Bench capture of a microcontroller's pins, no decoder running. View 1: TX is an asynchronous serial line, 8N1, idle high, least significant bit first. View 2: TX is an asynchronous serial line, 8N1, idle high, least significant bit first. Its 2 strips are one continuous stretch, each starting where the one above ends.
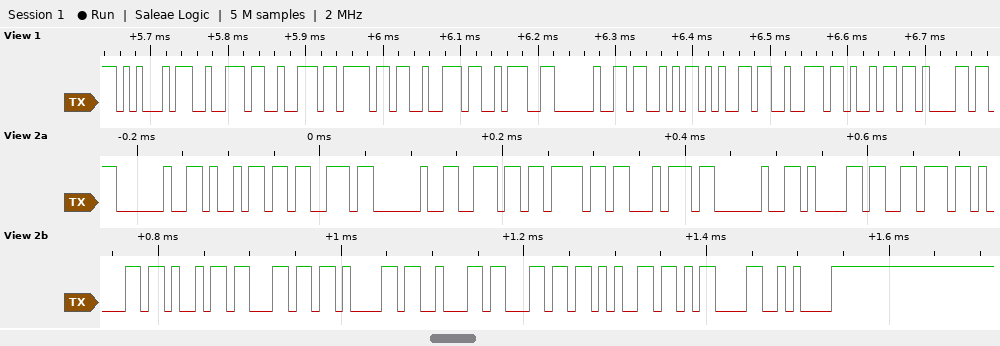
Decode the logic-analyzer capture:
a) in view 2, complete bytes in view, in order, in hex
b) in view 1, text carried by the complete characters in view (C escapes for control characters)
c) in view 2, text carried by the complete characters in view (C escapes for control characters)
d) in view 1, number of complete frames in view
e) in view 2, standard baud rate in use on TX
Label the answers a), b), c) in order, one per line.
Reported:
a) 20 69 73 20 6E 6F 74 20 61 76 61 69 6C 61 62 6C 65 0D 0A
b) "Error: Seria"
c) " is not available\r\n"
d) 12
e) 115200 baud
